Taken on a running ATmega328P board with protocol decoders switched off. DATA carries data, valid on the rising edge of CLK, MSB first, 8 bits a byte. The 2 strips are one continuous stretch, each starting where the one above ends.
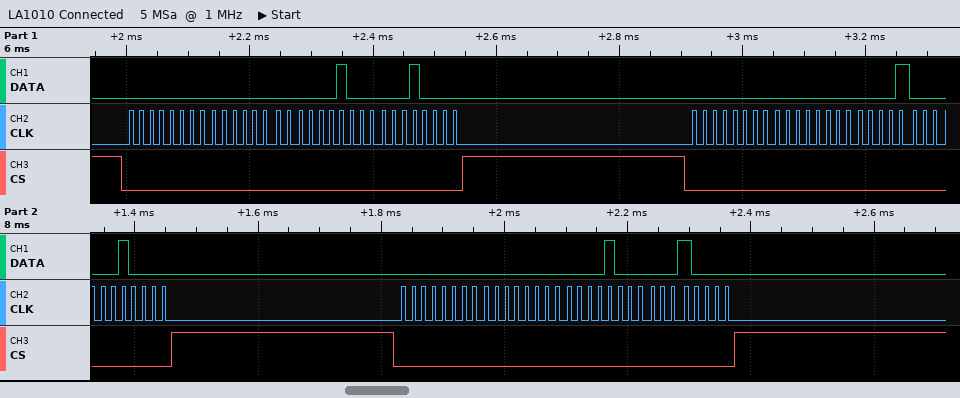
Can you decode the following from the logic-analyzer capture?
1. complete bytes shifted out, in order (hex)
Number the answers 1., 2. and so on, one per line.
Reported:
1. 0x00 0x00 0x08 0x10 0x00 0x00 0x08 0x10 0x00 0x00 0x08 0x10
